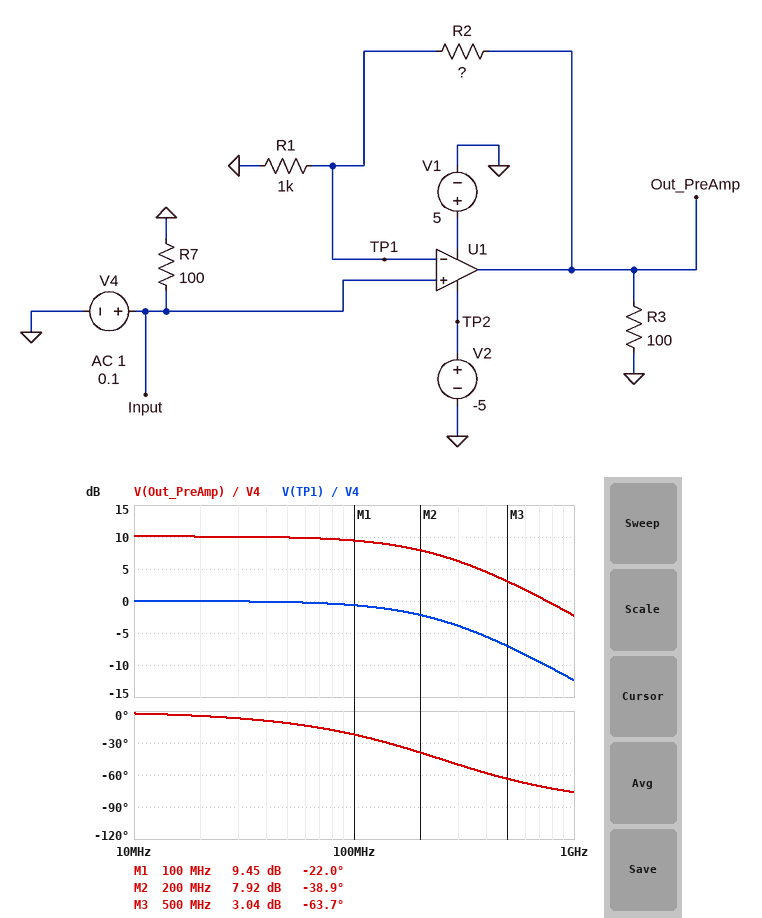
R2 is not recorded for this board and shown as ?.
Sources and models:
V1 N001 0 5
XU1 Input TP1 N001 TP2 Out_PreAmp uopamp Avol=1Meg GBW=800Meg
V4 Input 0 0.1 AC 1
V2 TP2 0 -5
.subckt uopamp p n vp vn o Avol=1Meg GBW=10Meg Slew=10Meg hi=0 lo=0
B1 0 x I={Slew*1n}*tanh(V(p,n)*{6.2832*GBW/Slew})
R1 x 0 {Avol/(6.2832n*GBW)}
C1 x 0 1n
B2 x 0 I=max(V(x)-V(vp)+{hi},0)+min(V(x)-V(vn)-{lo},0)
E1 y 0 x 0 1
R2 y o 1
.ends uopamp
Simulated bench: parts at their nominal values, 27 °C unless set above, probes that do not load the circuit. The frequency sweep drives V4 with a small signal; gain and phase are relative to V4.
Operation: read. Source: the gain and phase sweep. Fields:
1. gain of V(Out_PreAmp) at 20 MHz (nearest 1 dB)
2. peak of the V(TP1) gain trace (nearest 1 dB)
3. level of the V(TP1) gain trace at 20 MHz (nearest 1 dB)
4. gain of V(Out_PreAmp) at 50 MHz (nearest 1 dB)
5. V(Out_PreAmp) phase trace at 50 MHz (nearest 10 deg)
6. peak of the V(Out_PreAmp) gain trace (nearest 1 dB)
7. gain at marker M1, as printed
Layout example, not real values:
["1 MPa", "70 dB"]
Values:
["10 dB", "0 dB", "0 dB", "10 dB", "-10 deg", "10 dB", "9.45 dB"]
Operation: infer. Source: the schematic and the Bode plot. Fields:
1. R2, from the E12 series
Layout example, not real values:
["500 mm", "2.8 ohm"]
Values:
["2.2 kΩ"]
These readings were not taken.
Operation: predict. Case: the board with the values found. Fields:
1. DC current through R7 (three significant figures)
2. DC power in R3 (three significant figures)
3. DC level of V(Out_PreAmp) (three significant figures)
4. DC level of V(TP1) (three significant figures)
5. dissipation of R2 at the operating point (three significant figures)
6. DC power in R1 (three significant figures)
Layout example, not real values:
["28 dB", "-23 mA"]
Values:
["1.00 mA", "1.02 mW", "320 mV", "100 mV", "22.0 µW", "10.0 µW"]
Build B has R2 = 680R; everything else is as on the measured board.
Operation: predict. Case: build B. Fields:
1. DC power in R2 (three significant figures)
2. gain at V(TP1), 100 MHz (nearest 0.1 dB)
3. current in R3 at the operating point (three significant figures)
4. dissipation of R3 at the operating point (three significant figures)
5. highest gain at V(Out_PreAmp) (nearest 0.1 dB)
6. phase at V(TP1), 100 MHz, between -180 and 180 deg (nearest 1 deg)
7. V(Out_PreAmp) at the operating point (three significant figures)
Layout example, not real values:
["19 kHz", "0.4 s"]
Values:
["6.80 µW", "-0.2 dB", "1.68 mA", "282 µW", "4.5 dB", "-12 deg", "168 mV"]
